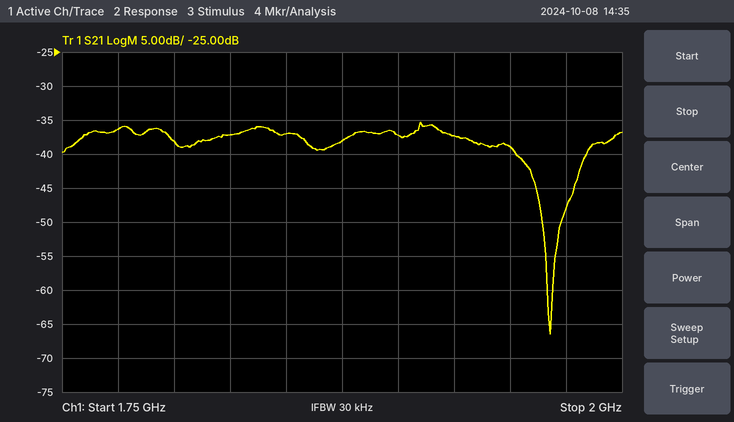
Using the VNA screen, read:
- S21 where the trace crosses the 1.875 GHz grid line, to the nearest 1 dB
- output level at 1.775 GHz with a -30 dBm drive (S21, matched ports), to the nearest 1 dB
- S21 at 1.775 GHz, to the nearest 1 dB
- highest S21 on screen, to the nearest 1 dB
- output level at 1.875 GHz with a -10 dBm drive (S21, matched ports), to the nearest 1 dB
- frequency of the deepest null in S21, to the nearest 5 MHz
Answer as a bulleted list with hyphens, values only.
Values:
- -38 dB
- -66 dBm
- -36 dB
- -35 dB
- -48 dBm
- 1.970 GHz
